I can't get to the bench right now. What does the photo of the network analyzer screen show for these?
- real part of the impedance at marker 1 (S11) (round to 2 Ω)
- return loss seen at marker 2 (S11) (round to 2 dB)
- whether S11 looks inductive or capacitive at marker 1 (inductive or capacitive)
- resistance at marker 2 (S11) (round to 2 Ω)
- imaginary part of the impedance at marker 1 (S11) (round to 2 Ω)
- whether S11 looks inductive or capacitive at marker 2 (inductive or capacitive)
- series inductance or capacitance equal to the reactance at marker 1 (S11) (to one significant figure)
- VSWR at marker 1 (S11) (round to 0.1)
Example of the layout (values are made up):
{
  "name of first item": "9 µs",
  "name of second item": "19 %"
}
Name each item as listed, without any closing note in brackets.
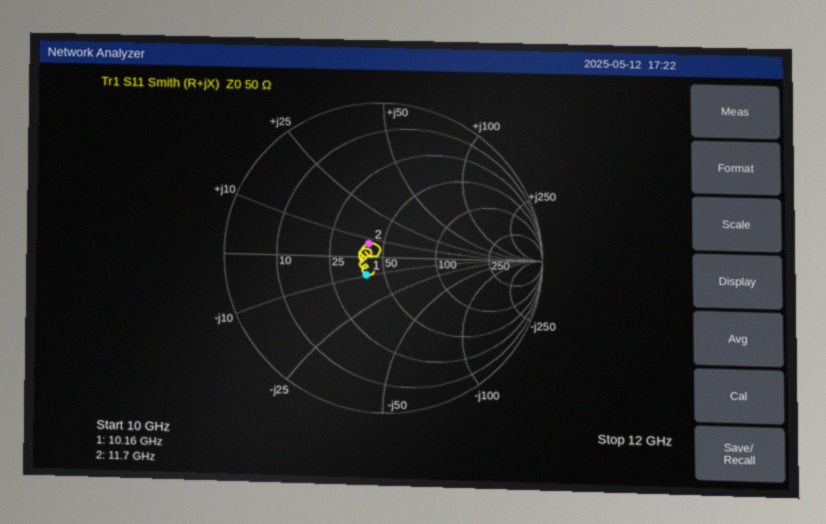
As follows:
{
  "real part of the impedance at marker 1 (S11)": "40 Ω",
  "return loss seen at marker 2 (S11)": "18 dB",
  "whether S11 looks inductive or capacitive at marker 1": "capacitive",
  "resistance at marker 2 (S11)": "42 Ω",
  "imaginary part of the impedance at marker 1 (S11)": "-10 Ω",
  "whether S11 looks inductive or capacitive at marker 2": "inductive",
  "series inductance or capacitance equal to the reactance at marker 1 (S11)": "2 pF",
  "VSWR at marker 1 (S11)": "1.4"
}
